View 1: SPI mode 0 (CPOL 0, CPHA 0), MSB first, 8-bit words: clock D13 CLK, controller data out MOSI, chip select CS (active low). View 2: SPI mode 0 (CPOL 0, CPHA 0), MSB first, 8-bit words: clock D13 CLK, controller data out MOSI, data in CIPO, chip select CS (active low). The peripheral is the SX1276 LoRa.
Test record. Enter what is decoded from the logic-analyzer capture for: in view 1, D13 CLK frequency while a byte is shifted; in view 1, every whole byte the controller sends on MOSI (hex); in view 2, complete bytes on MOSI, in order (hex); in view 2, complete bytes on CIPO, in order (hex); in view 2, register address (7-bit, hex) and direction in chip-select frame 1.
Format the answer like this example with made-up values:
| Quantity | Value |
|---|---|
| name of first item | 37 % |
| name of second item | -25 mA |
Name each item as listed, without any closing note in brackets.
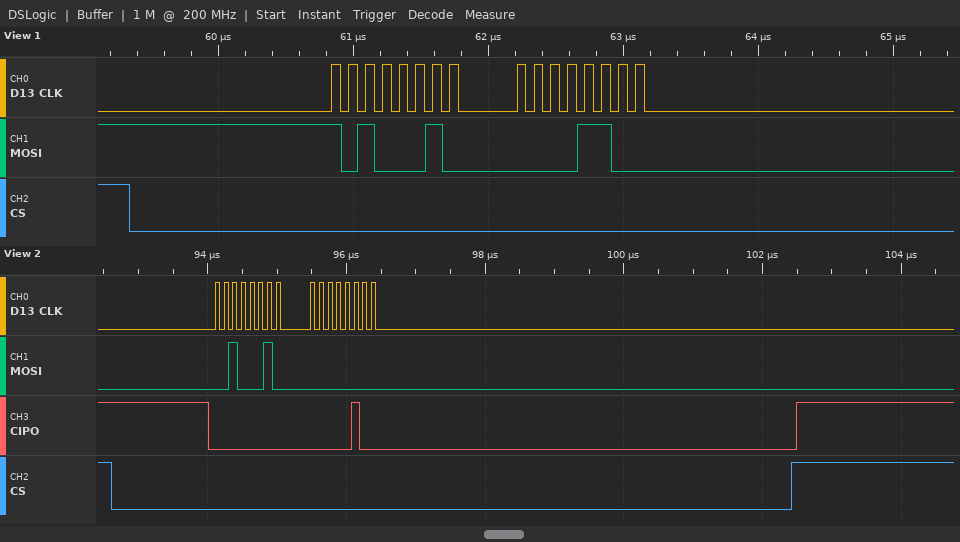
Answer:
| Quantity | Value |
|---|---|
| in view 1, D13 CLK frequency while a byte is shifted | 8 MHz |
| in view 1, every whole byte the controller sends on MOSI | A2 0C |
| in view 2, complete bytes on MOSI, in order | 0x22 0x00 |
| in view 2, complete bytes on CIPO, in order | 0x00 0x04 |
| in view 2, register address (7-bit, hex) and direction in chip-select frame 1 | 0x22 read |
